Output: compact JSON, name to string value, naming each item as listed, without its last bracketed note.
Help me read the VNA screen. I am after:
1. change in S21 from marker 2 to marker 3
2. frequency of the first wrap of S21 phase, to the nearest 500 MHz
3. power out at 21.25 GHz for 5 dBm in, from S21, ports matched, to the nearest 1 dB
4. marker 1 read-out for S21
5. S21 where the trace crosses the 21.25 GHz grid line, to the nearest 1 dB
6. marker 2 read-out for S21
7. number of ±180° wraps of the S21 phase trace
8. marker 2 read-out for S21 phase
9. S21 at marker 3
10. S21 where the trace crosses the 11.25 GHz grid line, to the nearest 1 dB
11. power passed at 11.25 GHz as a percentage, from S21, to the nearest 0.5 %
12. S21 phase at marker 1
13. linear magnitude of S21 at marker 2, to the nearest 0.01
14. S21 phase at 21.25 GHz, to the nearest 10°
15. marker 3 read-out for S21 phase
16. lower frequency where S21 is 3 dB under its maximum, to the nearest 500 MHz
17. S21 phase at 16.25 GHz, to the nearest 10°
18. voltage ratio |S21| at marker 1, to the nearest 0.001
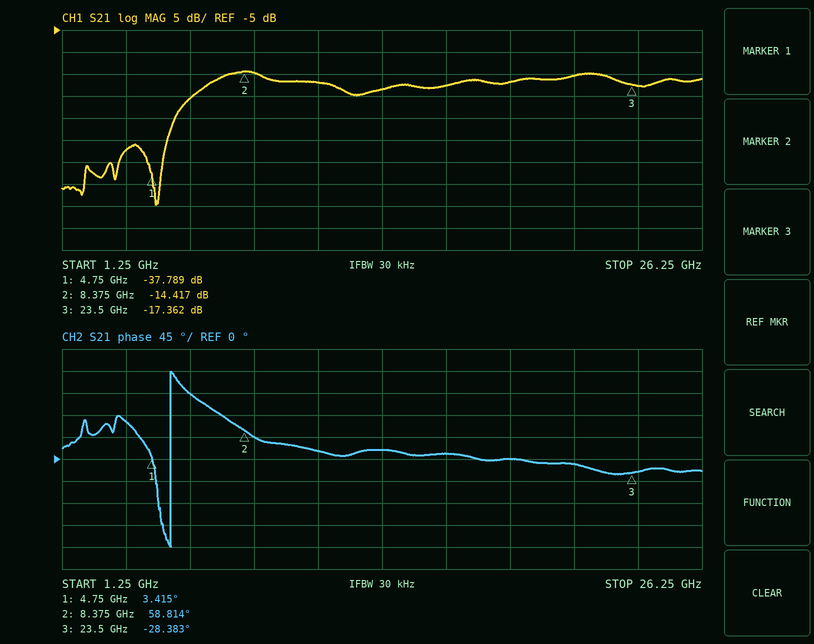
{"change in S21 from marker 2 to marker 3": "-2.945 dB", "frequency of the first wrap of S21 phase, to the nearest 500 MHz": "5.5 GHz", "power out at 21.25 GHz for 5 dBm in, from S21, ports matched, to the nearest 1 dB": "-10 dBm", "marker 1 read-out for S21": "-37.789 dB", "S21 where the trace crosses the 21.25 GHz grid line, to the nearest 1 dB": "-15 dB", "marker 2 read-out for S21": "-14.417 dB", "number of ±180° wraps of the S21 phase trace": "1", "marker 2 read-out for S21 phase": "58.814°", "S21 at marker 3": "-17.362 dB", "S21 where the trace crosses the 11.25 GHz grid line, to the nearest 1 dB": "-17 dB", "power passed at 11.25 GHz as a percentage, from S21, to the nearest 0.5 %": "2.0 %", "S21 phase at marker 1": "3.415°", "linear magnitude of S21 at marker 2, to the nearest 0.01": "0.19", "S21 phase at 21.25 GHz, to the nearest 10°": "-10°", "marker 3 read-out for S21 phase": "-28.383°", "lower frequency where S21 is 3 dB under its maximum, to the nearest 500 MHz": "7.0 GHz", "S21 phase at 16.25 GHz, to the nearest 10°": "10°", "voltage ratio |S21| at marker 1, to the nearest 0.001": "0.013"}
